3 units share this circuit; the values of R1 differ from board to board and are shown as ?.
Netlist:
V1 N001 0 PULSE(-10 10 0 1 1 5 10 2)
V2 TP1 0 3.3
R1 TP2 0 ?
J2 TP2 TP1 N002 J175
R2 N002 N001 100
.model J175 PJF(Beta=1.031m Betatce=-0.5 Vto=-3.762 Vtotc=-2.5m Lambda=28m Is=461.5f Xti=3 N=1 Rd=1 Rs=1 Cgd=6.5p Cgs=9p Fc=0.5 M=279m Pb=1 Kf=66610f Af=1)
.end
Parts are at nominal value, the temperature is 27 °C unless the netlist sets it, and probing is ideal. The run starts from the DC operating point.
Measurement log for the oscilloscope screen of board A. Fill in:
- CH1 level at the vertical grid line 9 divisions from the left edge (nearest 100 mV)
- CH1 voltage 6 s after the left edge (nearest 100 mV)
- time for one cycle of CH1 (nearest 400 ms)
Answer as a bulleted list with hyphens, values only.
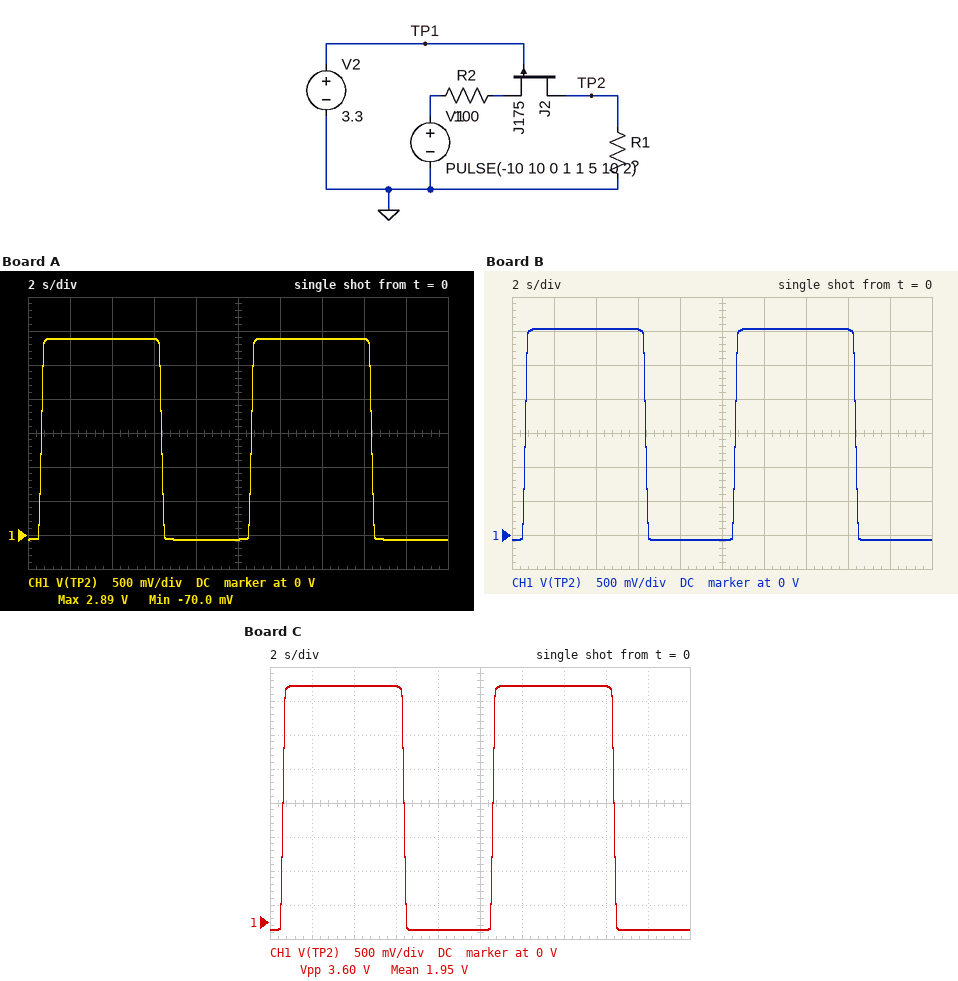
- -100 mV
- 2.9 V
- 10.0 s
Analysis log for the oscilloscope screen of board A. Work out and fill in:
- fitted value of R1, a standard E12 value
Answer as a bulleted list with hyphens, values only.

- 330 Ω
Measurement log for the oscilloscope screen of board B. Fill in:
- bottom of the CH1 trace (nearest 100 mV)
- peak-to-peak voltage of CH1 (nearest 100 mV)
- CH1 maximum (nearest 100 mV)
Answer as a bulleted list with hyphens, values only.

- -100 mV
- 3.1 V
- 3.0 V
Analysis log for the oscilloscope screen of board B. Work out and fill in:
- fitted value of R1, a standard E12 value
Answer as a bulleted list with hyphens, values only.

- 390 Ω
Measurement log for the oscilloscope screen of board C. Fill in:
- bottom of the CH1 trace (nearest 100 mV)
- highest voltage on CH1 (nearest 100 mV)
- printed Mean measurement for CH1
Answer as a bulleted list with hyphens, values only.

- -100 mV
- 3.5 V
- 1.95 V
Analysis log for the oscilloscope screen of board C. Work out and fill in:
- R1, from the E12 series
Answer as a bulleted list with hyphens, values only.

- 820 Ω
